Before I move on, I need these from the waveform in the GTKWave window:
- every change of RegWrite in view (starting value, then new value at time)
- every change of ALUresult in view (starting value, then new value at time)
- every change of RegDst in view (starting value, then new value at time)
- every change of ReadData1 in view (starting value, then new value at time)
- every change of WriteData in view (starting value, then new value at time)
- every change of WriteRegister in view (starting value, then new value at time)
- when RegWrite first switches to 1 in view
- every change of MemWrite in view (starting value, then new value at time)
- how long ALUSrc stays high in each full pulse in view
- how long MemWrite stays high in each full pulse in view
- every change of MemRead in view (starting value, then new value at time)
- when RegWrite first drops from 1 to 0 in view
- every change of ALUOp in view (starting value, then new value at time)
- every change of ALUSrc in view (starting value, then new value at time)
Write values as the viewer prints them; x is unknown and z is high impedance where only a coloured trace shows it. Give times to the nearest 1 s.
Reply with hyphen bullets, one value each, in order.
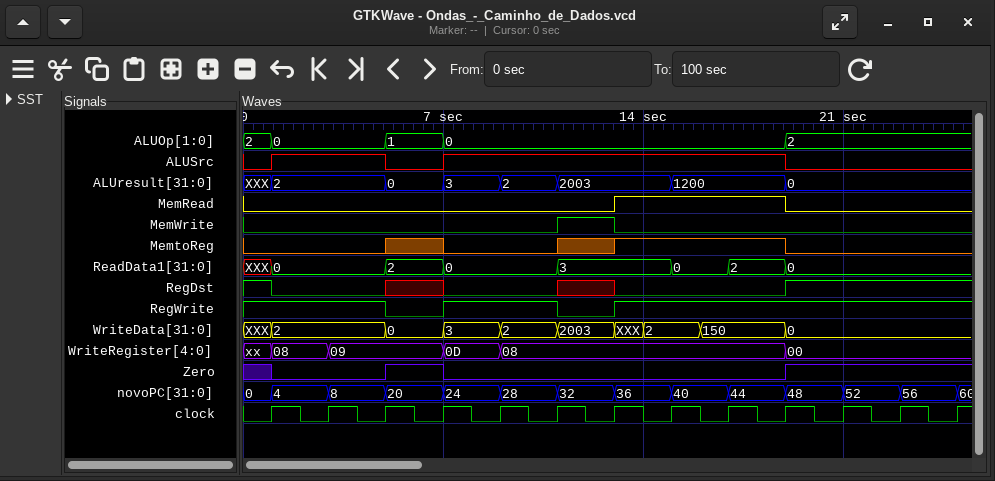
- 1, 0 at 5 s, 1 at 7 s, 0 at 11 s, 1 at 13 s
- XXX, 2 at 1 s, 0 at 5 s, 3 at 7 s, 2 at 9 s, 2003 at 11 s, 1200 at 15 s, 0 at 19 s
- 1, 0 at 1 s, x at 5 s, 0 at 7 s, x at 11 s, 0 at 13 s, 1 at 19 s
- XXX, 0 at 1 s, 2 at 5 s, 0 at 7 s, 3 at 11 s, 0 at 15 s, 2 at 17 s, 0 at 19 s
- XXX, 2 at 1 s, 0 at 5 s, 3 at 7 s, 2 at 9 s, 2003 at 11 s, XXX at 13 s, 2 at 14 s, 150 at 16 s, 0 at 19 s
- xx, 08 at 1 s, 09 at 3 s, 0D at 7 s, 08 at 9 s, 00 at 19 s
- 7 s
- 0, 1 at 11 s, 0 at 13 s
- 4 s, 12 s
- 2 s
- 0, 1 at 13 s, 0 at 19 s
- 5 s
- 2, 0 at 1 s, 1 at 5 s, 0 at 7 s, 2 at 19 s
- 0, 1 at 1 s, 0 at 5 s, 1 at 7 s, 0 at 19 s
